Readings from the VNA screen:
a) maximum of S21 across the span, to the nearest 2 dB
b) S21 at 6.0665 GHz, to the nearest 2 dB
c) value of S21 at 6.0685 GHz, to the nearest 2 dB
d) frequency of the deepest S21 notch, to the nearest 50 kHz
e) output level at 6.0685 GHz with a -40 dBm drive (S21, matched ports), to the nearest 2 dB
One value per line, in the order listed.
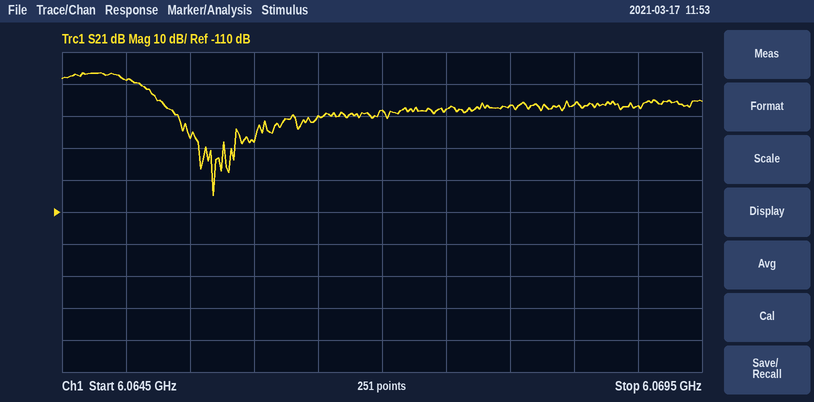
-66 dB
-80 dB
-76 dB
6.06570 GHz
-116 dBm
